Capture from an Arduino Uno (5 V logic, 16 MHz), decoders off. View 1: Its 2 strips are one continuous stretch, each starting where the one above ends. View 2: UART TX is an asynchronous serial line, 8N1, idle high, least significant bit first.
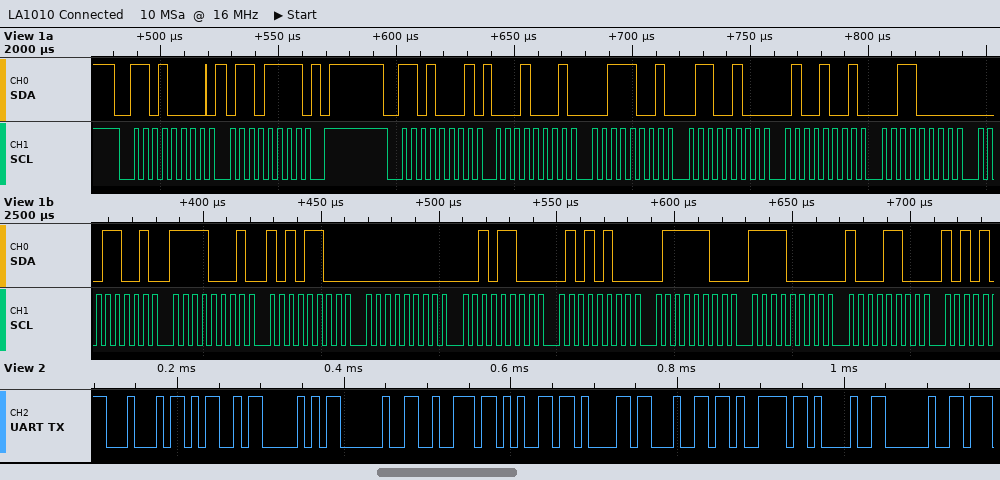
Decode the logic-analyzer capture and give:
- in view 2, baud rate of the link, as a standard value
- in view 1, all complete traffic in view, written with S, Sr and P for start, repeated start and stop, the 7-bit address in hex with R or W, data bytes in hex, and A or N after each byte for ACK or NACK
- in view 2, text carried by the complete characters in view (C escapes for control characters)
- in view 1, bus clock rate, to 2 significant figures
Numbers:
115200 baud
S 68W A 6F A P S 68R A 11 A 39 A 64 A 49 A 30 A 19 A F1 A AC A 00 A 2C A 54 A 7C A F0 A 8C A
"DMP ready! "
250 kHz
